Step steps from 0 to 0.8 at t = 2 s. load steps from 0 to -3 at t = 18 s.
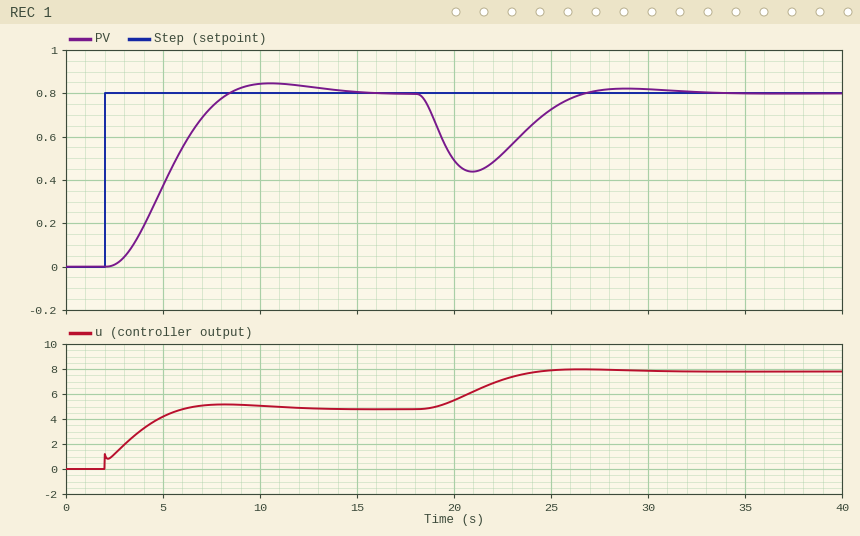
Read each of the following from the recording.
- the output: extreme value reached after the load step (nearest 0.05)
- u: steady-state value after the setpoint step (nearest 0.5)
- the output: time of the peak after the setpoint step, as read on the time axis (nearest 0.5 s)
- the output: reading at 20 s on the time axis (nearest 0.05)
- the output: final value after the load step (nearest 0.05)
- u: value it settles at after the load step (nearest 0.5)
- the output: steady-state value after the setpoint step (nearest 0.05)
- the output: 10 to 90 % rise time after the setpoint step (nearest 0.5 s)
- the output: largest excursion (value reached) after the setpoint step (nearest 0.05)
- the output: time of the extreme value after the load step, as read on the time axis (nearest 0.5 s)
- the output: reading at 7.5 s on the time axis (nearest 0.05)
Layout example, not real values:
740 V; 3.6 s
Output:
0.45; 5.0; 10.5 s; 0.50; 0.80; 8.0; 0.80; 4.0 s; 0.85; 21.0 s; 0.75
